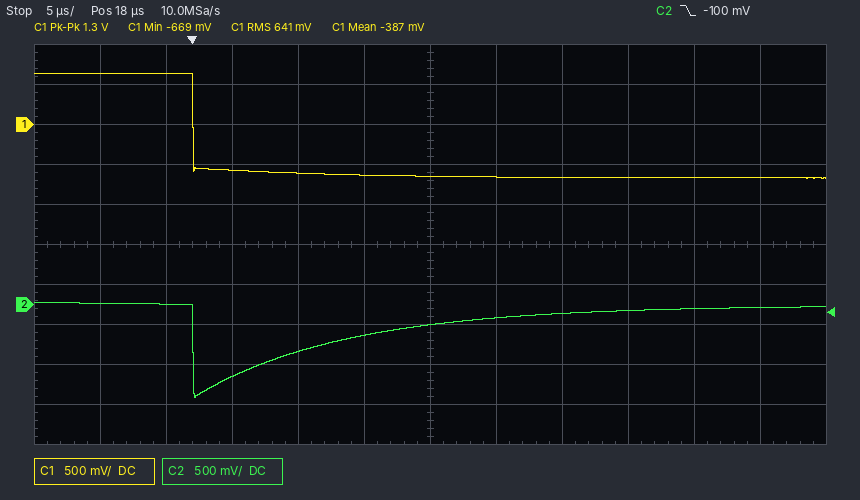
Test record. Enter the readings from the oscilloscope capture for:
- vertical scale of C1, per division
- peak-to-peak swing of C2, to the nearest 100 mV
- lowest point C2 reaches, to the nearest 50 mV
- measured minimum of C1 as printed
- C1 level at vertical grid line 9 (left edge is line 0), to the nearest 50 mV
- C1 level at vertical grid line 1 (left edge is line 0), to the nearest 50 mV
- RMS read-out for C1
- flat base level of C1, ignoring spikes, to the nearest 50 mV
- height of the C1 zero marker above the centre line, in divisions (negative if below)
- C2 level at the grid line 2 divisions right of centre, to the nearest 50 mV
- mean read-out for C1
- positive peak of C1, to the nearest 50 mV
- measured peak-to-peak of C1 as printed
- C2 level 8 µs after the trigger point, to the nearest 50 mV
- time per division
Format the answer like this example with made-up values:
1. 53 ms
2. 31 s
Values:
1. 500 mV
2. 1.20 V
3. -1.15 V
4. -669 mV
5. -650 mV
6. 650 mV
7. 641 mV
8. -650 mV
9. +3.0 div
10. -100 mV
11. -387 mV
12. 650 mV
13. 1.3 V
14. -600 mV
15. 5 µs
